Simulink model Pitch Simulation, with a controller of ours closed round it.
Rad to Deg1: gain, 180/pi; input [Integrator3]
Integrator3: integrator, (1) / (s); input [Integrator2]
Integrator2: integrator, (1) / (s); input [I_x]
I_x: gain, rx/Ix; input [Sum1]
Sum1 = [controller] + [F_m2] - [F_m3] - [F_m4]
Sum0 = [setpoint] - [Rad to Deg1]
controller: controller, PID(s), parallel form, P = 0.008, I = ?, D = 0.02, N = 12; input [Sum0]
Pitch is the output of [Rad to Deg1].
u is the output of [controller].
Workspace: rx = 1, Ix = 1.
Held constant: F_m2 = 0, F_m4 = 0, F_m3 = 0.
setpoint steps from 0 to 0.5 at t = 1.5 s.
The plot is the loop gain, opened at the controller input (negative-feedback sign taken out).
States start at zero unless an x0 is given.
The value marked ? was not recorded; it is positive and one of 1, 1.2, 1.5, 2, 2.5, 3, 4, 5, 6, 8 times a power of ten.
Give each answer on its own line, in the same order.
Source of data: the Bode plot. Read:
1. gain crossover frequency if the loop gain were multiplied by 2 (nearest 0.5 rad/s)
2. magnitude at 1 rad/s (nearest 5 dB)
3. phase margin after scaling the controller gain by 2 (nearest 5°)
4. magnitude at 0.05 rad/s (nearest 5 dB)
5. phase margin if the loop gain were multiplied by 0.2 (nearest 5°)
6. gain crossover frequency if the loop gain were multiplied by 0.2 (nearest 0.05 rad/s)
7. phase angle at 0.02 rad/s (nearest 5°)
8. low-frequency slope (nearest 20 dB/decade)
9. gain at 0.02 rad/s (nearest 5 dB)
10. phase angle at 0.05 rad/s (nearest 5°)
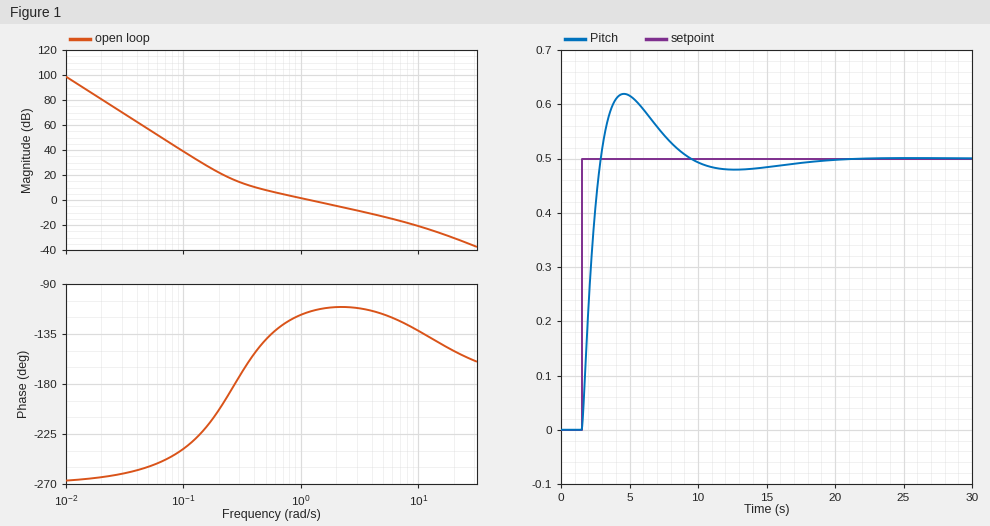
2.5 rad/s
0 dB
70°
55 dB
10°
0.30 rad/s
-265°
-60 dB/decade
80 dB
-255°
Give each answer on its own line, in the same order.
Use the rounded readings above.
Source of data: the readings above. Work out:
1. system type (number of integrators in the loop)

3
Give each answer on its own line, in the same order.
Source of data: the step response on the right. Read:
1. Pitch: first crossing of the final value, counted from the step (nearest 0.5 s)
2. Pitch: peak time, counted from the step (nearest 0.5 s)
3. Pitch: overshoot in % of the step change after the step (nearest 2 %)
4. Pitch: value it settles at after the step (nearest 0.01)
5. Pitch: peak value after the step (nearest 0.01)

1.5 s
3.0 s
24 %
0.50
0.62
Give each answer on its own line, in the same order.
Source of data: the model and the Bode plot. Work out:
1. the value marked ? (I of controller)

0.0015
